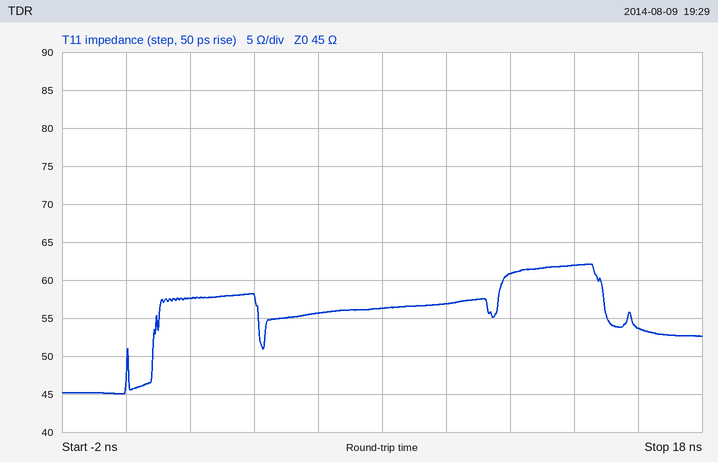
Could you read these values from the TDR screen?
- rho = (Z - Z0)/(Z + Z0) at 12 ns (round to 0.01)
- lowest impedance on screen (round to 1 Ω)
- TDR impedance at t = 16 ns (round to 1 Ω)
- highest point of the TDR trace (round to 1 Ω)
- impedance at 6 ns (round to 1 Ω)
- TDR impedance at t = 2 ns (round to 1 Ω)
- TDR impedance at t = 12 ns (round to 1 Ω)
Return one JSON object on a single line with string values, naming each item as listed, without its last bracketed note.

{"rho = (Z - Z0)/(Z + Z0) at 12 ns": "+0.15", "lowest impedance on screen": "45 Ω", "TDR impedance at t = 16 ns": "54 Ω", "highest point of the TDR trace": "62 Ω", "impedance at 6 ns": "56 Ω", "TDR impedance at t = 2 ns": "58 Ω", "TDR impedance at t = 12 ns": "61 Ω"}
